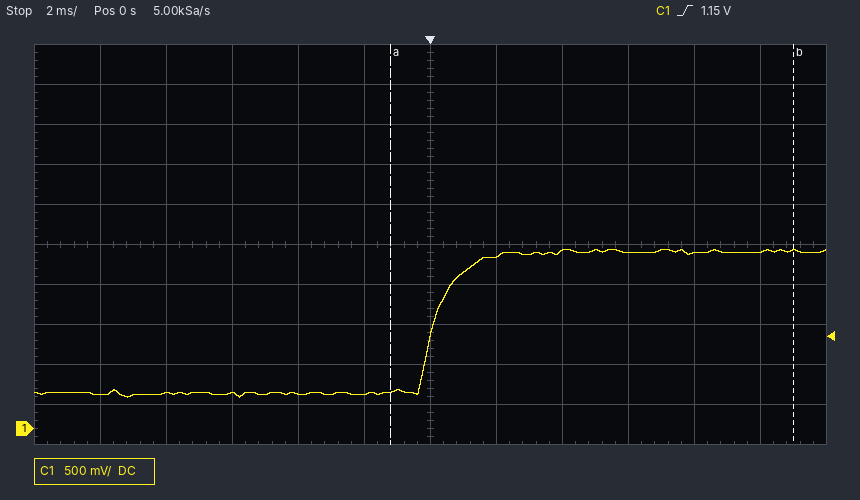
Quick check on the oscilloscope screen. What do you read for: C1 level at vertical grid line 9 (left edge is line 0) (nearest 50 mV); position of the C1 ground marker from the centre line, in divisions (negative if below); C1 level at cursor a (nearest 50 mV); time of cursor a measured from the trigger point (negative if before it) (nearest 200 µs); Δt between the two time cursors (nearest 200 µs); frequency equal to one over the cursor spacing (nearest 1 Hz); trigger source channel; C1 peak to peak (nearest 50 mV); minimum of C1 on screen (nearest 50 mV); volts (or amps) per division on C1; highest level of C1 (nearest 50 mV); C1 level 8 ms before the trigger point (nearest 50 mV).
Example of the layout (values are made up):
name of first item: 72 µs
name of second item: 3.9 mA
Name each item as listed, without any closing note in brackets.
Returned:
C1 level at vertical grid line 9 (left edge is line 0): 2.20 V
position of the C1 ground marker from the centre line, in divisions: -4.6 div
C1 level at cursor a: 450 mV
time of cursor a measured from the trigger point (negative if before it): -1.2 ms
Δt between the two time cursors: 12.2 ms
frequency equal to one over the cursor spacing: 82 Hz
trigger source channel: C1
C1 peak to peak: 1.85 V
minimum of C1 on screen: 400 mV
volts (or amps) per division on C1: 500 mV
highest level of C1: 2.25 V
C1 level 8 ms before the trigger point: 450 mV
